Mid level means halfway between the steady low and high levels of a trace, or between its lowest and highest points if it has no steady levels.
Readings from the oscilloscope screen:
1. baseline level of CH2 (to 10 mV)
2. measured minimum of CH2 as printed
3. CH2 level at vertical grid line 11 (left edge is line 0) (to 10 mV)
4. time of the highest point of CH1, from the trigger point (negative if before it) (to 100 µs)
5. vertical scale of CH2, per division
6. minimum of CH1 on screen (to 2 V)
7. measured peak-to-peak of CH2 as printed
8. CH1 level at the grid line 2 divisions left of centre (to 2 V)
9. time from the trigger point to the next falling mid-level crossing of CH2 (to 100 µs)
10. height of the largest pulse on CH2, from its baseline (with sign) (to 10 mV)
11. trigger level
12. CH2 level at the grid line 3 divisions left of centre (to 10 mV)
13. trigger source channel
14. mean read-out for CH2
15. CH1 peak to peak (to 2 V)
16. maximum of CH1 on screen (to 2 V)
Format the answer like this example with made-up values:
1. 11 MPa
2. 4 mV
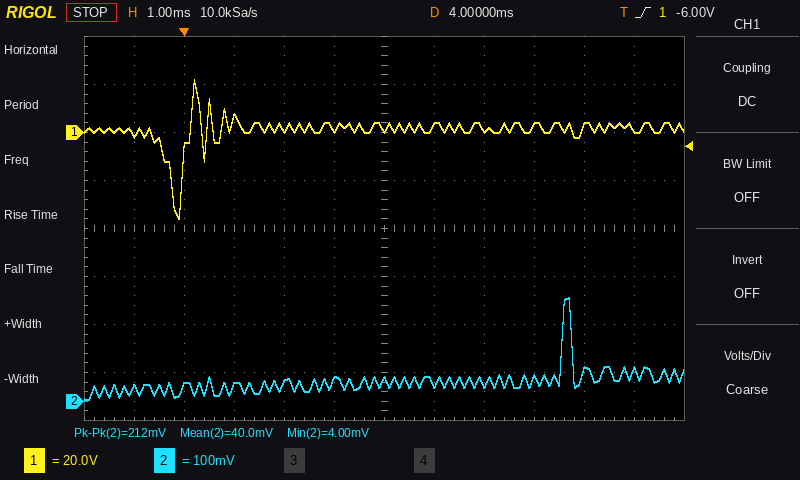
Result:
1. 40 mV
2. 4.00 mV
3. 60 mV
4. +200 µs
5. 100 mV
6. -36 V
7. 212 mV
8. 2 V
9. 7.8 ms
10. +180 mV
11. -6.00 V
12. 30 mV
13. CH1
14. 40.0 mV
15. 58 V
16. 22 V
